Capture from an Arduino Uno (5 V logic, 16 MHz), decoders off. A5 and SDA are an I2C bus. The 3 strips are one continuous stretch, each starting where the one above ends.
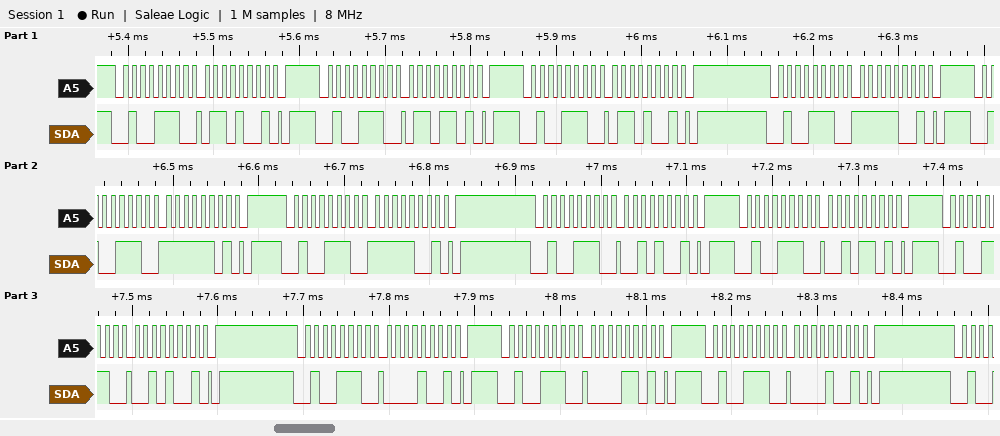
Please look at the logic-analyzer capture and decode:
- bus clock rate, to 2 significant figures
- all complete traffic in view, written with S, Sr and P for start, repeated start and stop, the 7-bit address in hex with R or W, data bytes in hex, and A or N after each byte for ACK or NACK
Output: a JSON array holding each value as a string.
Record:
["100 kHz", "S 27W A 69 A P S 27W A 6D A P S 27W A 69 A P S 27W A F9 A P S 27W A FD A P S 27W A F9 A P S 27W A 29 A P S 27W A 2D A P S 27W A 29 A P S 27W A 09 A P S 27W A 0D A P S 27W A 09 A P"]
